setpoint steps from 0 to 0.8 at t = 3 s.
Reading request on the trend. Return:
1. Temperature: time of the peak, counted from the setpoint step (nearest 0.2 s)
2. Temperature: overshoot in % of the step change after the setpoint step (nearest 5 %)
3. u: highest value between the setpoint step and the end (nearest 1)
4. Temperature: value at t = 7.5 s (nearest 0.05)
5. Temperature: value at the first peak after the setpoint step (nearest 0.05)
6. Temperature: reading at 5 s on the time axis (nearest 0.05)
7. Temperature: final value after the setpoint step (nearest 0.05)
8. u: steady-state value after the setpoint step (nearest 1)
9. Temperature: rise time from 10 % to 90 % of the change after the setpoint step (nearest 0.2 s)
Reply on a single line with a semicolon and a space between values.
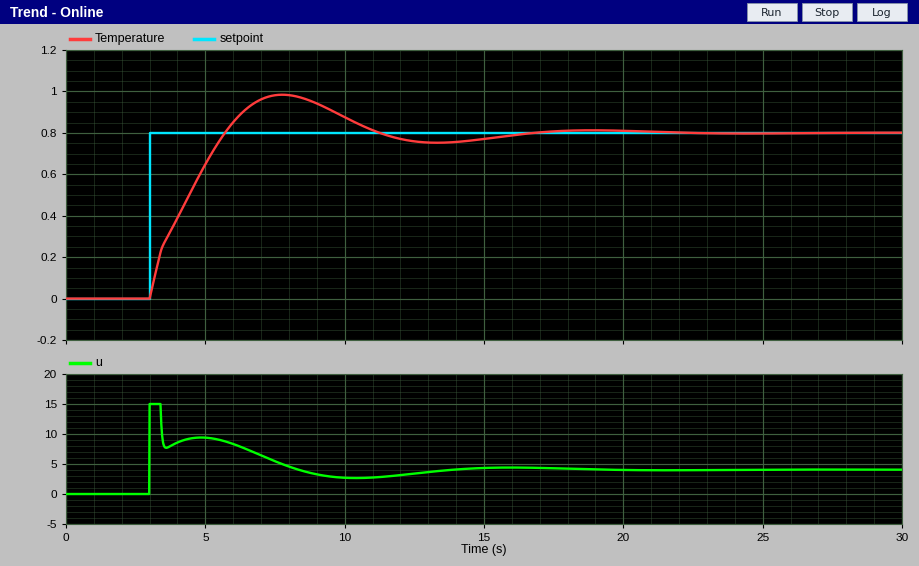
4.8 s; 25 %; 15; 1.00; 1.00; 0.65; 0.80; 4; 2.2 s
